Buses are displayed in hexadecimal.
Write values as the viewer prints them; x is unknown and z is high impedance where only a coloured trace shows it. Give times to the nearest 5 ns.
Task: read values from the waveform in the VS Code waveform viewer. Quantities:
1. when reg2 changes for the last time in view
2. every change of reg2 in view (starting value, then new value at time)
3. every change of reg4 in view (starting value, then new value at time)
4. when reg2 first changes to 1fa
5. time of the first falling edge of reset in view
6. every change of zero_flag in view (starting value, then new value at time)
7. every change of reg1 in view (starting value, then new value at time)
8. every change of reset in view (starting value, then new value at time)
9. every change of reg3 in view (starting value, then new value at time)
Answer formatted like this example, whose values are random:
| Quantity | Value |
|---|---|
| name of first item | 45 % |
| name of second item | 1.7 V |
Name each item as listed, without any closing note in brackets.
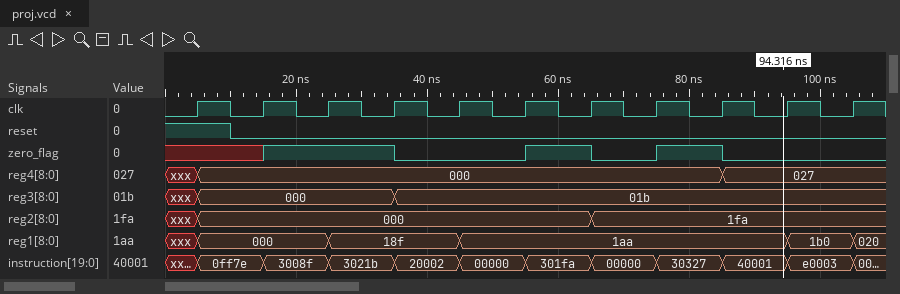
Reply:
| Quantity | Value |
|---|---|
| when reg2 changes for the last time in view | 65 ns |
| every change of reg2 in view | xxx, 000 at 5 ns, 1fa at 65 ns |
| every change of reg4 in view | xxx, 000 at 5 ns, 027 at 85 ns |
| when reg2 first changes to 1fa | 65 ns |
| time of the first falling edge of reset in view | 10 ns |
| every change of zero_flag in view | x, 1 at 15 ns, 0 at 35 ns, 1 at 55 ns, 0 at 65 ns, 1 at 75 ns, 0 at 85 ns |
| every change of reg1 in view | xxx, 000 at 5 ns, 18f at 25 ns, 1aa at 45 ns, 1b0 at 95 ns, 020 at 105 ns |
| every change of reset in view | 1, 0 at 10 ns |
| every change of reg3 in view | xxx, 000 at 5 ns, 01b at 35 ns |
